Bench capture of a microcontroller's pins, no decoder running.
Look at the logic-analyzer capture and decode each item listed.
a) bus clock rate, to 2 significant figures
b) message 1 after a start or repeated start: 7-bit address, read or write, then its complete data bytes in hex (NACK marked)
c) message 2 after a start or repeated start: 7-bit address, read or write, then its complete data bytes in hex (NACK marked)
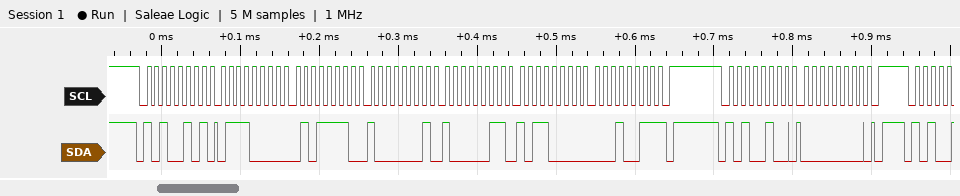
100 kHz
0x52 read: 70 5E 81 83 B0 13 NACK
0x52 write: 00
